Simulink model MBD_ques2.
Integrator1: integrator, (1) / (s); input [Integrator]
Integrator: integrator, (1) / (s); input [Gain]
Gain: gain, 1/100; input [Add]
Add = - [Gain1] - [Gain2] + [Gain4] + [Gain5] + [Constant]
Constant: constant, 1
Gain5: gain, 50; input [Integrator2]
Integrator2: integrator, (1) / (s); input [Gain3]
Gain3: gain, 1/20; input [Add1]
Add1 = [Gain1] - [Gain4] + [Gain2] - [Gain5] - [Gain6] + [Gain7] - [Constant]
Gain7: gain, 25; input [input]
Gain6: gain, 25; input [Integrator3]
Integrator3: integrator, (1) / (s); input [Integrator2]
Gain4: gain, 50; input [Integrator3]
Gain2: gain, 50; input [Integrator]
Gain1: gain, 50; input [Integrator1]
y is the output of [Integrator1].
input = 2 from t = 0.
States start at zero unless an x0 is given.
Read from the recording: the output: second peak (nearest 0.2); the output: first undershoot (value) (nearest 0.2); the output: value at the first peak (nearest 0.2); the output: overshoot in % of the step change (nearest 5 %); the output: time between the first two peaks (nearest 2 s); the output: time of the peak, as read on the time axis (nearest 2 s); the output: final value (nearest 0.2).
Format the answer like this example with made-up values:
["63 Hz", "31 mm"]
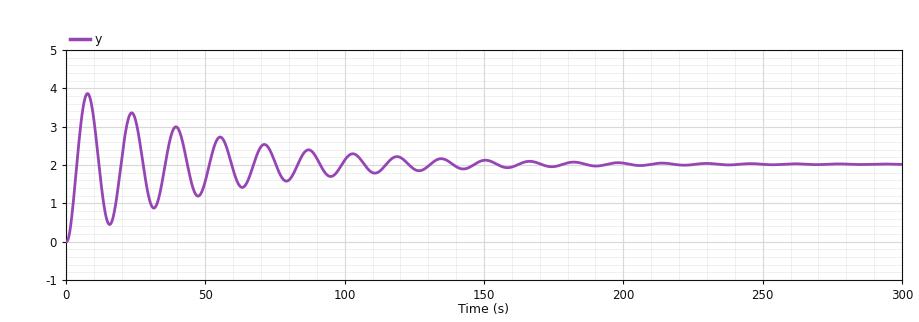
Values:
["3.4", "0.4", "3.8", "90 %", "16 s", "8 s", "2.0"]
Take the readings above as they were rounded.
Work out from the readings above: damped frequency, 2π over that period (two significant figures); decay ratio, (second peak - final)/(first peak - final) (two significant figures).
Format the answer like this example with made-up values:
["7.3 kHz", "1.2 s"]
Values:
["0.39 rad/s", "0.78"]
